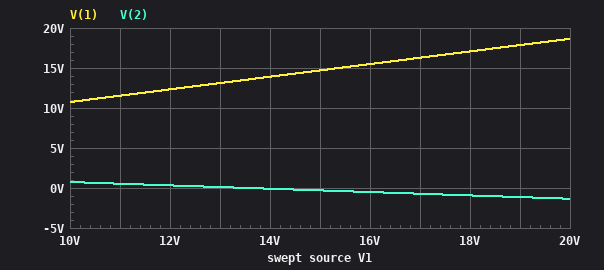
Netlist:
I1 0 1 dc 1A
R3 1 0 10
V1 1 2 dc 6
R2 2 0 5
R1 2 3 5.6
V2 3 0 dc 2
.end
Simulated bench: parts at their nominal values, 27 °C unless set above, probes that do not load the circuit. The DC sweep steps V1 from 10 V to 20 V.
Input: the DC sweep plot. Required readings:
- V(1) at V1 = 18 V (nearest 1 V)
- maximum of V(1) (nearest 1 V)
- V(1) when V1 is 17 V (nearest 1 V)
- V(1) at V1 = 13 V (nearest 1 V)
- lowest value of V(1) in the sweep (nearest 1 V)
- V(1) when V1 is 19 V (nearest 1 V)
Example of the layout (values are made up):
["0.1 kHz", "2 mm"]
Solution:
["17 V", "19 V", "16 V", "13 V", "11 V", "18 V"]
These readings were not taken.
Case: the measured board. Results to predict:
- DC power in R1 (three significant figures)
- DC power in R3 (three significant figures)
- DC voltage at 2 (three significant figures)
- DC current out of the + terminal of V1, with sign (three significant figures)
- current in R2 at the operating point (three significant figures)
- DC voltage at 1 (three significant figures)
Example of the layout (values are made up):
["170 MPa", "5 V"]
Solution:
["31.2 mW", "5.75 W", "1.58 V", "-242 mA", "316 mA", "7.58 V"]
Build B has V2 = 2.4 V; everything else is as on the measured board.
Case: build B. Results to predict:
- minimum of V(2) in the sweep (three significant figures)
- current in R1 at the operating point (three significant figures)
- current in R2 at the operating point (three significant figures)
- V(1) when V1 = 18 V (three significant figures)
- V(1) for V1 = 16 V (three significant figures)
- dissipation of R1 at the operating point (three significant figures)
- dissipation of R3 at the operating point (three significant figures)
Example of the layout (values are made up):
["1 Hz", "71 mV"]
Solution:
["-1.19 V", "119 mA", "346 mA", "17.2 V", "15.6 V", "79.8 mW", "5.98 W"]
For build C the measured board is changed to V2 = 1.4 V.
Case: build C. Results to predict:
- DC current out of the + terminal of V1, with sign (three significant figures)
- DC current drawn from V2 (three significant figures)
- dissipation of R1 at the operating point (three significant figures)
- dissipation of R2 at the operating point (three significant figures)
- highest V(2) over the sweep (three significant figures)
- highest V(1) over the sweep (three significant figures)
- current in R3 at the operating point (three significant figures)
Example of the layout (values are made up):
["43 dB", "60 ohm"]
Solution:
["-264 mA", "7.46 mA", "312 µW", "369 mW", "522 mV", "18.4 V", "736 mA"]
